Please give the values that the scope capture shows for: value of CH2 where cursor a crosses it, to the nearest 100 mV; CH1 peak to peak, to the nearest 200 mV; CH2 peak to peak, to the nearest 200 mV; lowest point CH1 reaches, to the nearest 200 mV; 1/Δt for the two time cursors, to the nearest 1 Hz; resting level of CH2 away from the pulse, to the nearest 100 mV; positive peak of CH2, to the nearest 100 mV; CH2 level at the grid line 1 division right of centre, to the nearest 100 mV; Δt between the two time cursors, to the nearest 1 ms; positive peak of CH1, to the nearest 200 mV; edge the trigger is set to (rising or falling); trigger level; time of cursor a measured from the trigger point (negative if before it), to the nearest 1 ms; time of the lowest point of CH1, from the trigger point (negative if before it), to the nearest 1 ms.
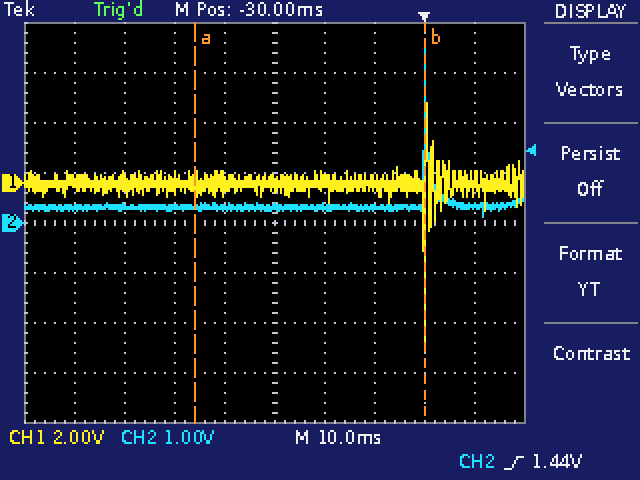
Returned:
300 mV
9.6 V
3.4 V
-6.4 V
22 Hz
300 mV
3.5 V
300 mV
46 ms
3.2 V
rising
1.44 V
-46 ms
0 ms
